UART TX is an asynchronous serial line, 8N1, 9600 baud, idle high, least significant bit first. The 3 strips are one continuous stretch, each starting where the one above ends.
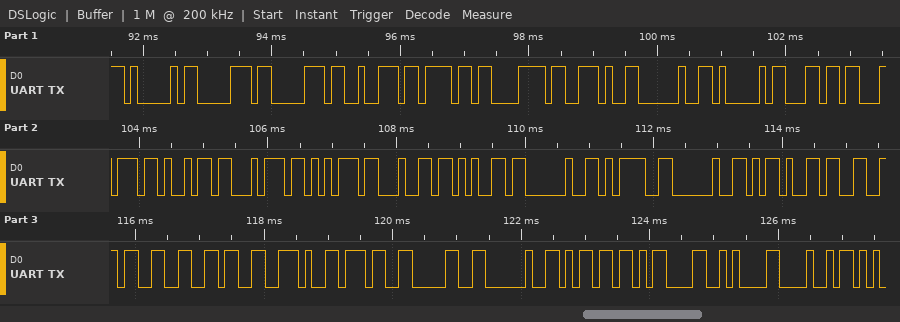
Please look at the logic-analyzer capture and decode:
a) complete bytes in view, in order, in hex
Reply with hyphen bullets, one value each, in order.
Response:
- 41 70 70 72 6F 78 2E 20 41 6C 74 69 74 75 64 65 20 3D 20 2D 33 33 36 2E 37 30 20 6D 0D 0A 48
